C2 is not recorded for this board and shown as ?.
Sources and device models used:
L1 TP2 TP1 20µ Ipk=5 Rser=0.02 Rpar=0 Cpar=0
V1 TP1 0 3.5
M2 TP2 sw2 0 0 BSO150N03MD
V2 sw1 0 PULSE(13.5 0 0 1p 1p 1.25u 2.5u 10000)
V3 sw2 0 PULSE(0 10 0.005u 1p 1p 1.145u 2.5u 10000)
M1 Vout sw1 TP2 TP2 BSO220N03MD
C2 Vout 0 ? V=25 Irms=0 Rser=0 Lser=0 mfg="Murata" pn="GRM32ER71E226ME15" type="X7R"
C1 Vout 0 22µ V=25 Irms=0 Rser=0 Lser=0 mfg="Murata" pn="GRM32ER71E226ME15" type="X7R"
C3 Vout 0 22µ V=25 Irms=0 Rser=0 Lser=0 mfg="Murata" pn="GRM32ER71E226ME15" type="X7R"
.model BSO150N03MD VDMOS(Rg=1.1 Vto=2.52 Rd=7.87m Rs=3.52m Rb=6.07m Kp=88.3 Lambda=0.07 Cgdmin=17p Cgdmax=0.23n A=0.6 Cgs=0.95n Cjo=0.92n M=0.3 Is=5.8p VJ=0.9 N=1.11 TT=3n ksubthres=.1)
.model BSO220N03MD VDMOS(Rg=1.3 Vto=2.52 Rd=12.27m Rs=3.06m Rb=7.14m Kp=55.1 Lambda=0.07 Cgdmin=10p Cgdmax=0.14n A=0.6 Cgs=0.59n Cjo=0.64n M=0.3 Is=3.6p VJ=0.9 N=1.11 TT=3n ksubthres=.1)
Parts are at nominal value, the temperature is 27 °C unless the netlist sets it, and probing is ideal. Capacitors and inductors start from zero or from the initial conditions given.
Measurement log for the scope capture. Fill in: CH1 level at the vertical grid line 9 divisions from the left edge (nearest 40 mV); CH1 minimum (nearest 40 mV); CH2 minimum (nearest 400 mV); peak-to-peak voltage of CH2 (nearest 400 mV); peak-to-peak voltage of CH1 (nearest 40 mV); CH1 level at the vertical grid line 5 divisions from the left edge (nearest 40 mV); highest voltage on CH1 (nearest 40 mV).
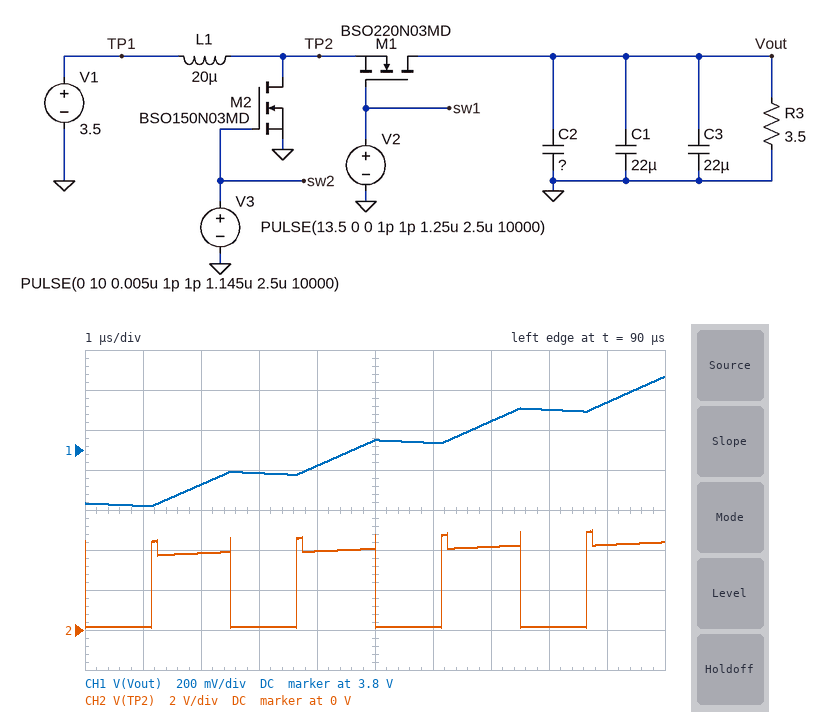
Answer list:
4.04 V
3.52 V
0 V
4.8 V
640 mV
3.84 V
4.16 V
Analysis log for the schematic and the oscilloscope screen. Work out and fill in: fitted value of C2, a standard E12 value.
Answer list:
39 µF
